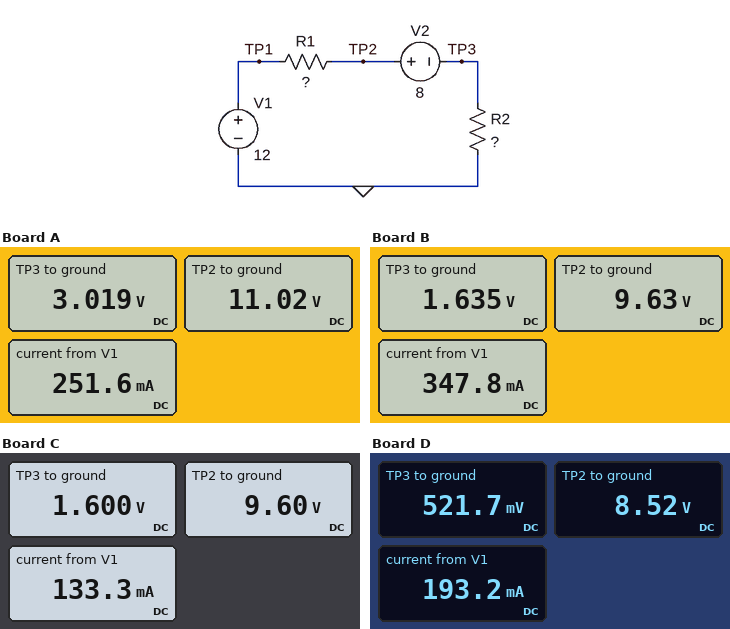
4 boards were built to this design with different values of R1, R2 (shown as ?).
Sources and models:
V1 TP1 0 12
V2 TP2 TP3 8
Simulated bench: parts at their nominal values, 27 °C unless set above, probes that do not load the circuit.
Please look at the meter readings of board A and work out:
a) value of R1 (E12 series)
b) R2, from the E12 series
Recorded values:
3.9 Ω
12 Ω
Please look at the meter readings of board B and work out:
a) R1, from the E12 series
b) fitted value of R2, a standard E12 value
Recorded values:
6.8 Ω
4.7 Ω
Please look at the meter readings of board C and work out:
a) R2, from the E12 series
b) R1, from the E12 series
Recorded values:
12 Ω
18 Ω
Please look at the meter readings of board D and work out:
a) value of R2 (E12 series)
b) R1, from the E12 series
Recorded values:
2.7 Ω
18 Ω
